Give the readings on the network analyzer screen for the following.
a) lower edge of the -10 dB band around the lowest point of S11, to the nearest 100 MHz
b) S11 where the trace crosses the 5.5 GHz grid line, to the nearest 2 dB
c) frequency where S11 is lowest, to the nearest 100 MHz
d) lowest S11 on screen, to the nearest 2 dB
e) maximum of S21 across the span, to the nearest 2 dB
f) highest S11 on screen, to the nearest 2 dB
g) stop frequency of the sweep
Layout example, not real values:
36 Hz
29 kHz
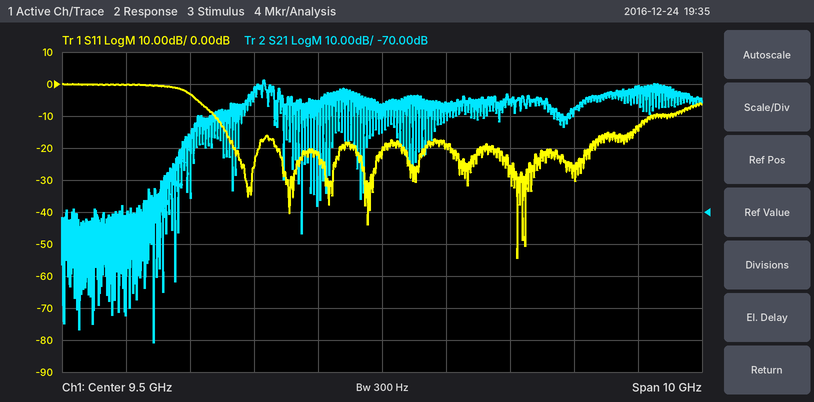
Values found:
6.9 GHz
0 dB
11.6 GHz
-54 dB
-28 dB
0 dB
14.5 GHz
